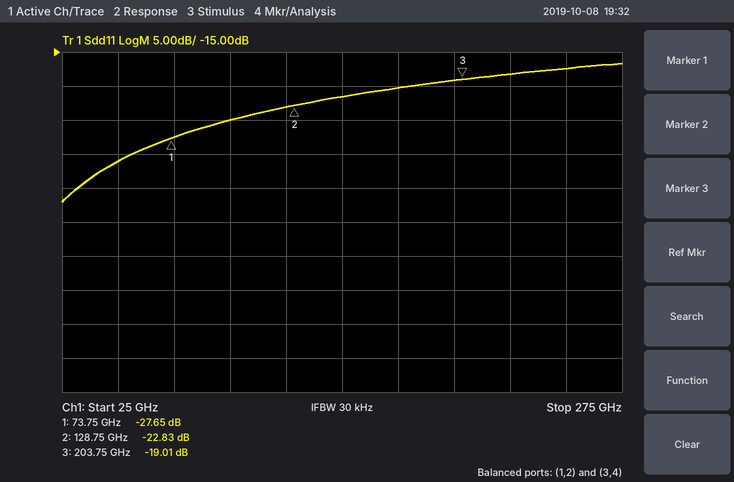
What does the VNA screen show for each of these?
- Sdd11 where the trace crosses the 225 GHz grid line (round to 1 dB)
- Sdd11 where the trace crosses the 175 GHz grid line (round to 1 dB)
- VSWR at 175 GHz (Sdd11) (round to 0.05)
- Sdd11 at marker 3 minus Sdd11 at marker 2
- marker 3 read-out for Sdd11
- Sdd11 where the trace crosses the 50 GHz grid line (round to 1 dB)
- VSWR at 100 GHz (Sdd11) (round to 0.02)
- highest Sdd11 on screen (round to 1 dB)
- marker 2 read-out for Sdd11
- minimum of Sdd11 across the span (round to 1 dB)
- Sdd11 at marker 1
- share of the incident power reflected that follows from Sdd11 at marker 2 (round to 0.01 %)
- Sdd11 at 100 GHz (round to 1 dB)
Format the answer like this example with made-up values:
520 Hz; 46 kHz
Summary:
-18 dB; -20 dB; 1.20; 3.82 dB; -19.01 dB; -31 dB; 1.12; -17 dB; -22.83 dB; -37 dB; -27.65 dB; 0.52 %; -25 dB
